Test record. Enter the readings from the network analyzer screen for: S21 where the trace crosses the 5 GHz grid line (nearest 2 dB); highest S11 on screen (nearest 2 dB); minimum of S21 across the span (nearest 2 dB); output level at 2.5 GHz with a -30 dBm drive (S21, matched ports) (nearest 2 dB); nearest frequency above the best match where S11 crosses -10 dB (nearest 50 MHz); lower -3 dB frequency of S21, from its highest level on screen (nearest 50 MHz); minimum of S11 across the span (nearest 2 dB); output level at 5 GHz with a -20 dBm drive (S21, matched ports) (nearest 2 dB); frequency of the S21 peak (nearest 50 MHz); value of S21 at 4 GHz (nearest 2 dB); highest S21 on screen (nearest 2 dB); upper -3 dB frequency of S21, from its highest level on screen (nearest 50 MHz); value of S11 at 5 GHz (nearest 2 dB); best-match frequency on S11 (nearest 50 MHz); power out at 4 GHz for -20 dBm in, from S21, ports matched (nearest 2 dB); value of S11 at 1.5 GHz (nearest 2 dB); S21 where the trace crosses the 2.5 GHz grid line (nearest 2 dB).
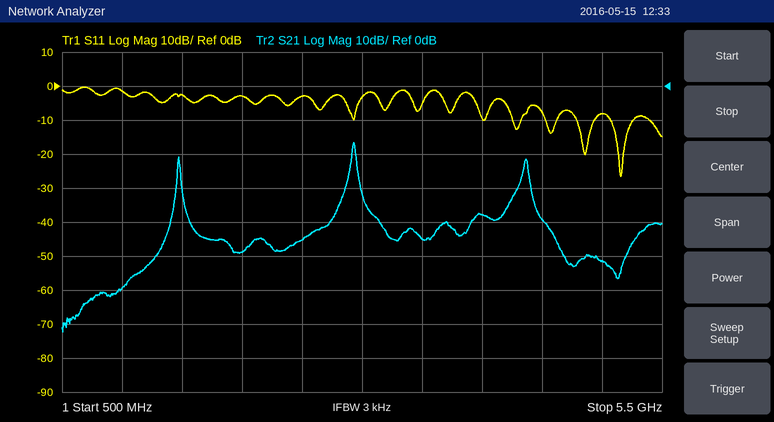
-52 dB
0 dB
-72 dB
-76 dBm
5.25 GHz
2.90 GHz
-26 dB
-72 dBm
2.95 GHz
-38 dB
-16 dB
2.95 GHz
-8 dB
5.15 GHz
-58 dBm
-2 dB
-46 dB
